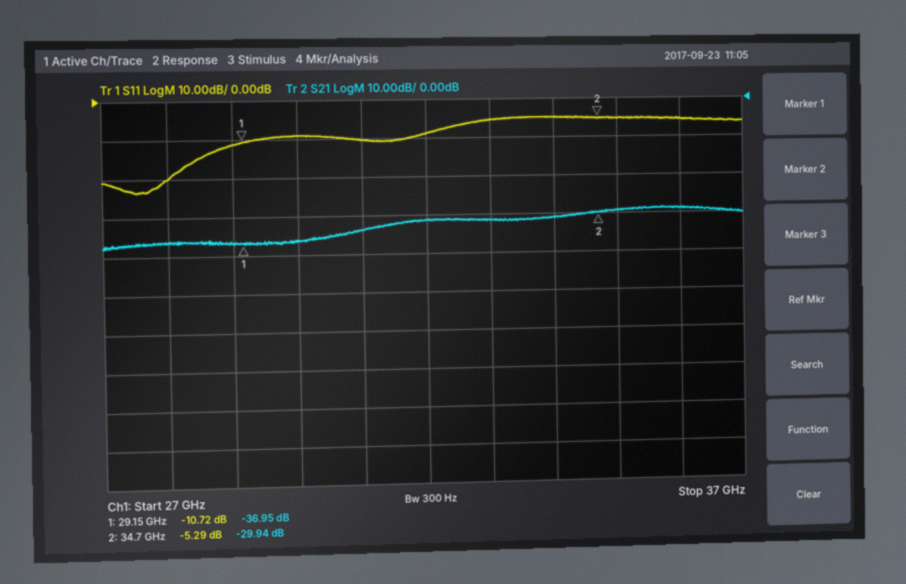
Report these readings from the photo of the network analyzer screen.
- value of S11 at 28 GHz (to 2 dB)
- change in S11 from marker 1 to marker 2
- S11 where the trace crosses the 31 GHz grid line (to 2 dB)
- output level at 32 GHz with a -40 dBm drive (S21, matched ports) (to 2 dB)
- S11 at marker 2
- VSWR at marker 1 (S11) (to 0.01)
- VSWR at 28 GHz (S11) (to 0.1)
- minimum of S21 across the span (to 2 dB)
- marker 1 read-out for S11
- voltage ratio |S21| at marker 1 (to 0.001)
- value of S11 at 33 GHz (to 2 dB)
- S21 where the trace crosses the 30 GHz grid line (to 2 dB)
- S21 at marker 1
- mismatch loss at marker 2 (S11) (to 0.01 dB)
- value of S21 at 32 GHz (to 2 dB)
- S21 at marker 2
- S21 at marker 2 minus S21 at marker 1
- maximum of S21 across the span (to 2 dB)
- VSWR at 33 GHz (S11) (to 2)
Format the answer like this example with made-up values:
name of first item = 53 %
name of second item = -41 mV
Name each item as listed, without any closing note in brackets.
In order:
value of S11 at 28 GHz = -20 dB
change in S11 from marker 1 to marker 2 = 5.43 dB
S11 where the trace crosses the 31 GHz grid line = -10 dB
output level at 32 GHz with a -40 dBm drive (S21, matched ports) = -72 dBm
S11 at marker 2 = -5.29 dB
VSWR at marker 1 (S11) = 1.82
VSWR at 28 GHz (S11) = 1.2
minimum of S21 across the span = -38 dB
marker 1 read-out for S11 = -10.72 dB
voltage ratio |S21| at marker 1 = 0.014
value of S11 at 33 GHz = -6 dB
S21 where the trace crosses the 30 GHz grid line = -36 dB
S21 at marker 1 = -36.95 dB
mismatch loss at marker 2 (S11) = 1.52 dB
value of S21 at 32 GHz = -32 dB
S21 at marker 2 = -29.94 dB
S21 at marker 2 minus S21 at marker 1 = 7.01 dB
maximum of S21 across the span = -28 dB
VSWR at 33 GHz (S11) = 4
